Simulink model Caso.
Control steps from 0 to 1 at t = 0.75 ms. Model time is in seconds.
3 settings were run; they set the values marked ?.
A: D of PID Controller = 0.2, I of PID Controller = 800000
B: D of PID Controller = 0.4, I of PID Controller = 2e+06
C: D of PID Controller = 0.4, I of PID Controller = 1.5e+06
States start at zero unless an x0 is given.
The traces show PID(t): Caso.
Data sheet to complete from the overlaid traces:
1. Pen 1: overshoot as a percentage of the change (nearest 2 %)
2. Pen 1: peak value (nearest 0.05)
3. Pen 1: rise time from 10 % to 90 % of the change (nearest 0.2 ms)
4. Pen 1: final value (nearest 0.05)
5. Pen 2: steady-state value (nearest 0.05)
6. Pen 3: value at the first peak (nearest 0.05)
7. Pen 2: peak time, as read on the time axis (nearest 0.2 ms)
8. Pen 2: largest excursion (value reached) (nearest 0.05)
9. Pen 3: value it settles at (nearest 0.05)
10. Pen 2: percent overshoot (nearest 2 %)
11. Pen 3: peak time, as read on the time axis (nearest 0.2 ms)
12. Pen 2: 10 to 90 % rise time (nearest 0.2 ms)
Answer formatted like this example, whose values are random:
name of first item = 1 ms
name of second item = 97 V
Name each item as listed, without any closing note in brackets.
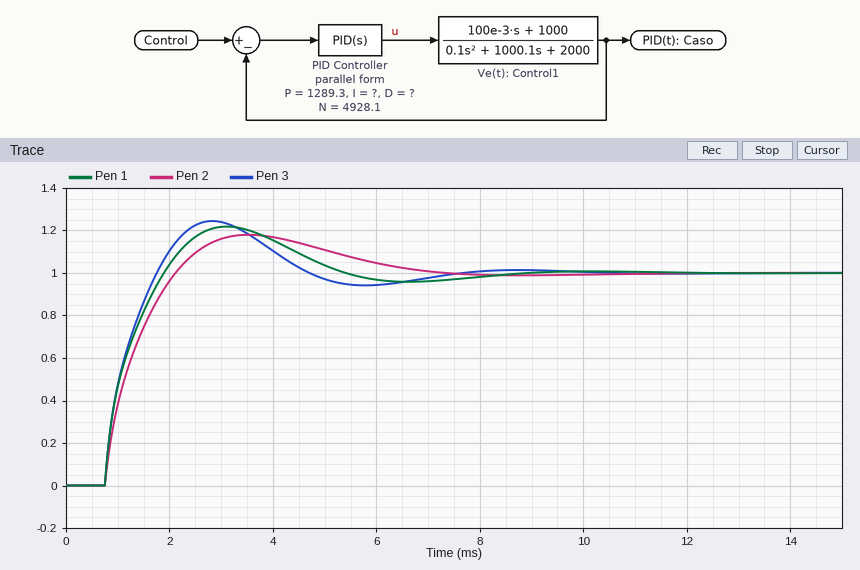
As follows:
Pen 1: overshoot as a percentage of the change = 22 %
Pen 1: peak value = 1.20
Pen 1: rise time from 10 % to 90 % of the change = 0.8 ms
Pen 1: final value = 1.00
Pen 2: steady-state value = 1.00
Pen 3: value at the first peak = 1.25
Pen 2: peak time, as read on the time axis = 3.6 ms
Pen 2: largest excursion (value reached) = 1.20
Pen 3: value it settles at = 1.00
Pen 2: percent overshoot = 18 %
Pen 3: peak time, as read on the time axis = 2.8 ms
Pen 2: 10 to 90 % rise time = 1.0 ms
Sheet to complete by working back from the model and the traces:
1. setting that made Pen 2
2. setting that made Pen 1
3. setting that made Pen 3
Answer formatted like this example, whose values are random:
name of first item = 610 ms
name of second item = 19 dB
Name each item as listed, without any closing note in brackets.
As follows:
setting that made Pen 2 = A
setting that made Pen 1 = C
setting that made Pen 3 = B
